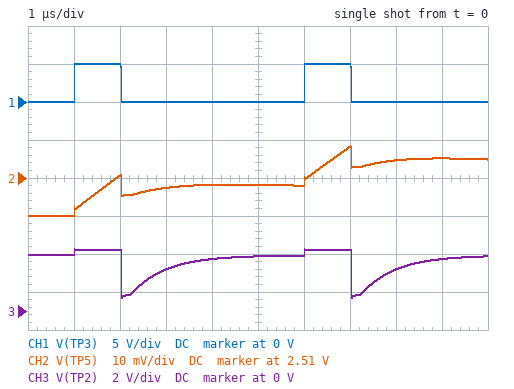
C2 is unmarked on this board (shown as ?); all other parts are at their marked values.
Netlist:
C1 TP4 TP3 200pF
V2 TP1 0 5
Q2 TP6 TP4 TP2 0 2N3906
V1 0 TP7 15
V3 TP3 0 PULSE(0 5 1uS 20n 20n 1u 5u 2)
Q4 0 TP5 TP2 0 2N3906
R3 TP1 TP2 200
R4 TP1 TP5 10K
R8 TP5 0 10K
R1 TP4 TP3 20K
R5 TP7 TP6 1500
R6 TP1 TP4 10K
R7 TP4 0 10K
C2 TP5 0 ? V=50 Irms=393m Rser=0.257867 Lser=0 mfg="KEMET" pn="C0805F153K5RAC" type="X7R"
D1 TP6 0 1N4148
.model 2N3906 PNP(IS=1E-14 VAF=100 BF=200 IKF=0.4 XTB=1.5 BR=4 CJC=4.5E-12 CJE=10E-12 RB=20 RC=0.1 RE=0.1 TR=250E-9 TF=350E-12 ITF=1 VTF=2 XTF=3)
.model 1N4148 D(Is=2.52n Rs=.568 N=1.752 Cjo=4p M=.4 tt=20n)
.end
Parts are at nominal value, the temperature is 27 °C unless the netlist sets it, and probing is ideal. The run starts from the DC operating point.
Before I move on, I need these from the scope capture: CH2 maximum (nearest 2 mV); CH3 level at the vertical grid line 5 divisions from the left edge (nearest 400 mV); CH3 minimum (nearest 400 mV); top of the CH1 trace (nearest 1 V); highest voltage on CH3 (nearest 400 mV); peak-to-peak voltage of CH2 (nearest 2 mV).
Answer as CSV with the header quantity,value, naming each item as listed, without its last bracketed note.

quantity,value
CH2 maximum,2.518 V
CH3 level at the vertical grid line 5 divisions from the left edge,2.8 V
CH3 minimum,800 mV
top of the CH1 trace,5 V
highest voltage on CH3,3.2 V
peak-to-peak voltage of CH2,18 mV
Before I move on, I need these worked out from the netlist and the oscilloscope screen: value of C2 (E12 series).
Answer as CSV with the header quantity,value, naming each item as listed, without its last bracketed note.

quantity,value
value of C2,4.7 nF
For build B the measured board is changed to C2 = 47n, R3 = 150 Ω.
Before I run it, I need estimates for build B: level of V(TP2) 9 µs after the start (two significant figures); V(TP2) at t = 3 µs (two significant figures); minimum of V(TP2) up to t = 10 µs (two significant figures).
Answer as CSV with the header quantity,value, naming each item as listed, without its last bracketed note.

quantity,value
level of V(TP2) 9 µs after the start,2.8 V
V(TP2) at t = 3 µs,2.3 V
minimum of V(TP2) up to t = 10 µs,770 mV
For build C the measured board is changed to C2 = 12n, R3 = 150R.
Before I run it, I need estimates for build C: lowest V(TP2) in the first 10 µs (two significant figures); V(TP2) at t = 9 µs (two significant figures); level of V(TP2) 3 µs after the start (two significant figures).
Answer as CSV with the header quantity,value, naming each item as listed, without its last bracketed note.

quantity,value
lowest V(TP2) in the first 10 µs,770 mV
V(TP2) at t = 9 µs,2.8 V
level of V(TP2) 3 µs after the start,2.3 V
